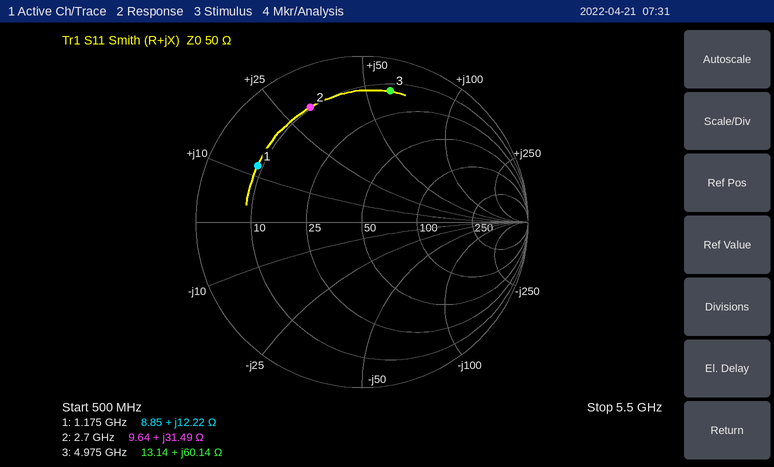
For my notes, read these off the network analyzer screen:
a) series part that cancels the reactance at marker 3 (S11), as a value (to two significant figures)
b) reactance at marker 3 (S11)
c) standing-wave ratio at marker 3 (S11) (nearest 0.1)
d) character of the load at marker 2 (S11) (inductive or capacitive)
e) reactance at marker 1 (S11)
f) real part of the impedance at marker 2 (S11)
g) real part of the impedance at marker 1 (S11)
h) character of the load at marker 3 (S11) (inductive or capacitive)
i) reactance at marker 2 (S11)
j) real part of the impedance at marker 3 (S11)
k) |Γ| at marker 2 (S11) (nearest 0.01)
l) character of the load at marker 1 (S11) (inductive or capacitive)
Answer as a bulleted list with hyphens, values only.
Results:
- 530 fF
- +60.14 Ω
- 9.5
- inductive
- +12.22 Ω
- 9.64 Ω
- 8.85 Ω
- inductive
- +31.49 Ω
- 13.14 Ω
- 0.76
- inductive
